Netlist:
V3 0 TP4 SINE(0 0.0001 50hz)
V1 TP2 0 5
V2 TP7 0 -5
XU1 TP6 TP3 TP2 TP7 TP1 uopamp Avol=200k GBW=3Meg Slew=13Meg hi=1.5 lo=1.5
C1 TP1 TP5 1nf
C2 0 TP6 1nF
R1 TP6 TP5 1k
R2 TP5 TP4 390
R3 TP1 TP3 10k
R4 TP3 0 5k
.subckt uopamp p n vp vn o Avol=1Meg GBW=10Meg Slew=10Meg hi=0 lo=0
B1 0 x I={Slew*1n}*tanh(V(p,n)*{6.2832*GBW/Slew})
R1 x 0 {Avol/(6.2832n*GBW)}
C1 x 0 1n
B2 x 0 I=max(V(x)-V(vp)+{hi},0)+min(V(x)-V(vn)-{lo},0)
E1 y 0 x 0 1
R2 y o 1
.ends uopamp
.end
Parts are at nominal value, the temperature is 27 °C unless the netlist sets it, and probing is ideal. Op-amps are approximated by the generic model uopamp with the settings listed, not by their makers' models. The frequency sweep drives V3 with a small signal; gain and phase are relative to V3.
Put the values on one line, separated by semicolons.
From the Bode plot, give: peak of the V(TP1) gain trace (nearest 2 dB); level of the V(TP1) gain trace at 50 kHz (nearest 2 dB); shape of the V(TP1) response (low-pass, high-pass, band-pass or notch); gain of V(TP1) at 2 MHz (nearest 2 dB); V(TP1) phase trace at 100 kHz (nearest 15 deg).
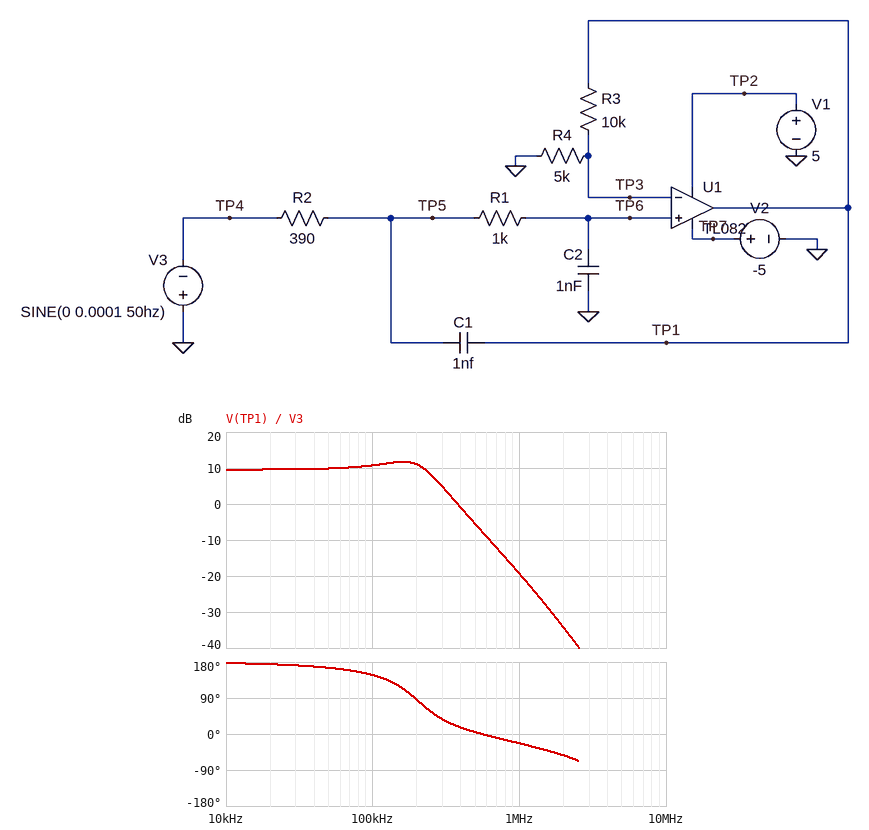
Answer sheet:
12 dB; 10 dB; low-pass; -34 dB; 150 deg
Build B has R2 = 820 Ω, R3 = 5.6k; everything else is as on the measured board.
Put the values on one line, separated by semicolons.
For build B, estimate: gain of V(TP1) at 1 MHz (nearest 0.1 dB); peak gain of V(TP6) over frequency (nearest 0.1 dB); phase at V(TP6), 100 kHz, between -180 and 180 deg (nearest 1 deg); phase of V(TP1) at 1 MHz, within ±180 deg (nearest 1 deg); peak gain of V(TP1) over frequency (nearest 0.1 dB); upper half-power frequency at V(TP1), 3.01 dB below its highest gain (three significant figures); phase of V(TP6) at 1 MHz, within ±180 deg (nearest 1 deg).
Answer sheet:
-26.8 dB; 1.8 dB; 136 deg; -22 deg; 8.3 dB; 185 kHz; 14 deg
